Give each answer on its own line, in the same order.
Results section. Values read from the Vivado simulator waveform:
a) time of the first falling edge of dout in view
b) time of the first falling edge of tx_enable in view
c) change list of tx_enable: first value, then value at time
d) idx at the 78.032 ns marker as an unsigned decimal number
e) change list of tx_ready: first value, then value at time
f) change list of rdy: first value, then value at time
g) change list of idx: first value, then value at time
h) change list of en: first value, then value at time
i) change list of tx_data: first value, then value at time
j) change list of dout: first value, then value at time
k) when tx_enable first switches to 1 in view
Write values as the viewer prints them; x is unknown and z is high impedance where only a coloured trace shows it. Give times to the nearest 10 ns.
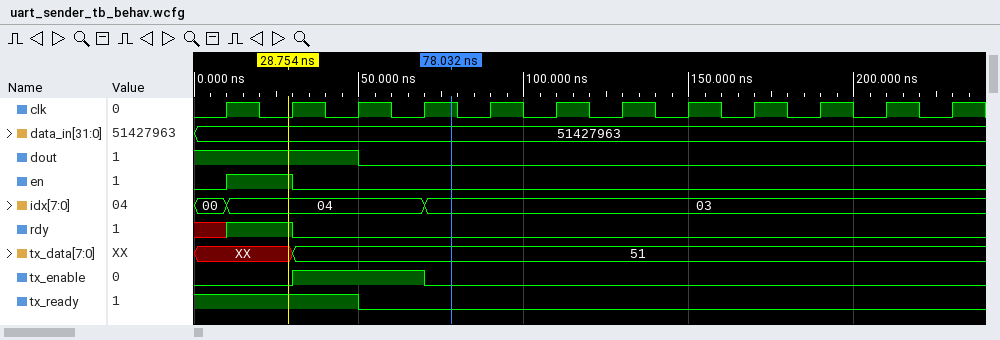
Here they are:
50 ns
70 ns
0, 1 at 30 ns, 0 at 70 ns
3
1, 0 at 50 ns
x, 1 at 10 ns, 0 at 30 ns
00, 04 at 10 ns, 03 at 70 ns
0, 1 at 10 ns, 0 at 30 ns
XX, 51 at 30 ns
1, 0 at 50 ns
30 ns
